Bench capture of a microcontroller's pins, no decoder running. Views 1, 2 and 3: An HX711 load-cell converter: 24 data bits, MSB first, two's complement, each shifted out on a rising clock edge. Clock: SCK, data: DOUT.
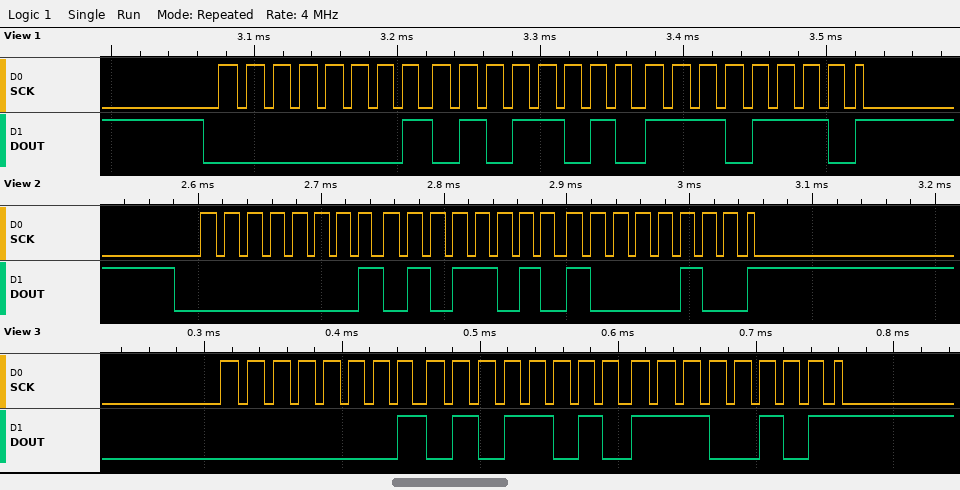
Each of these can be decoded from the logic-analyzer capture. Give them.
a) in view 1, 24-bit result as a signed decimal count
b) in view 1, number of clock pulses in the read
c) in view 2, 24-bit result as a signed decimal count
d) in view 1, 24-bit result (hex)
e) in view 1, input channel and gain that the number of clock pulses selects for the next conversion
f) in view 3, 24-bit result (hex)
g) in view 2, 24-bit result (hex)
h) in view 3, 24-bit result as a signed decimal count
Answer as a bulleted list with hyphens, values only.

- 88814
- 25
- 88708
- 0x015AEE
- channel A, gain 128
- 0x015AE5
- 0x015A84
- 88805
